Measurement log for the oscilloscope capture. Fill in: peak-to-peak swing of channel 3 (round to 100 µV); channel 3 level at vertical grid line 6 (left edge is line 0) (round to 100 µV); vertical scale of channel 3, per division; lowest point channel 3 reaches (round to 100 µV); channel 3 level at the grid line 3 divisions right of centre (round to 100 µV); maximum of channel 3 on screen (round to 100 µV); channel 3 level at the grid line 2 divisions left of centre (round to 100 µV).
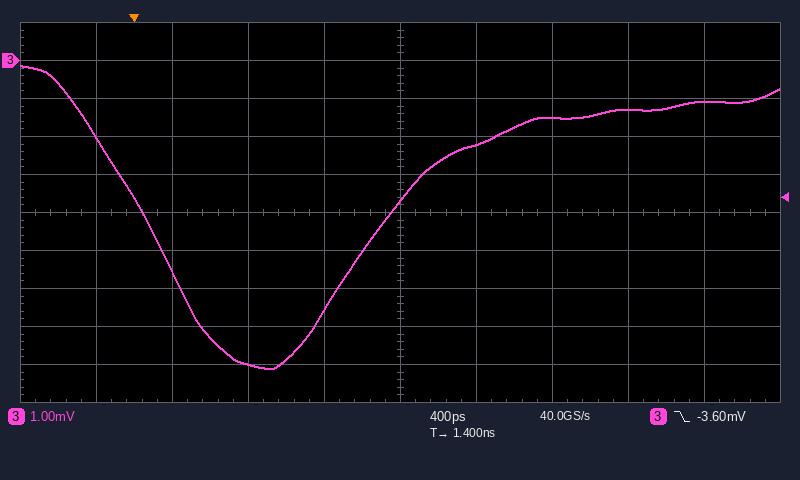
8.0 mV
-2.2 mV
1 mV
-8.1 mV
-1.3 mV
-100 µV
-8.0 mV
